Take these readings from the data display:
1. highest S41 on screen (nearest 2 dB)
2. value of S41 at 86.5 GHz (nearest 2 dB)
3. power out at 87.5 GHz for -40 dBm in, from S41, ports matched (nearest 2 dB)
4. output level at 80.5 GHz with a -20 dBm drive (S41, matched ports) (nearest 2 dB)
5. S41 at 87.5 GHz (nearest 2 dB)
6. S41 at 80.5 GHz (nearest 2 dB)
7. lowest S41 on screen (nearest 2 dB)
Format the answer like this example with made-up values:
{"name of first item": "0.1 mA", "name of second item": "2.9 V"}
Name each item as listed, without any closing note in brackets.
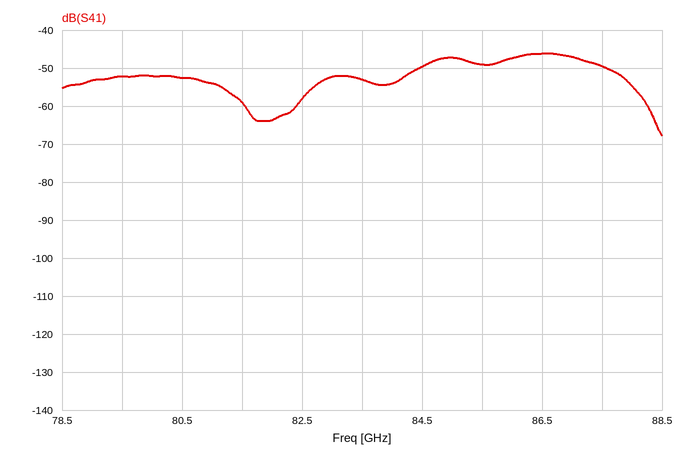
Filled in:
{"highest S41 on screen": "-46 dB", "value of S41 at 86.5 GHz": "-46 dB", "power out at 87.5 GHz for -40 dBm in, from S41, ports matched": "-90 dBm", "output level at 80.5 GHz with a -20 dBm drive (S41, matched ports)": "-72 dBm", "S41 at 87.5 GHz": "-50 dB", "S41 at 80.5 GHz": "-52 dB", "lowest S41 on screen": "-68 dB"}
